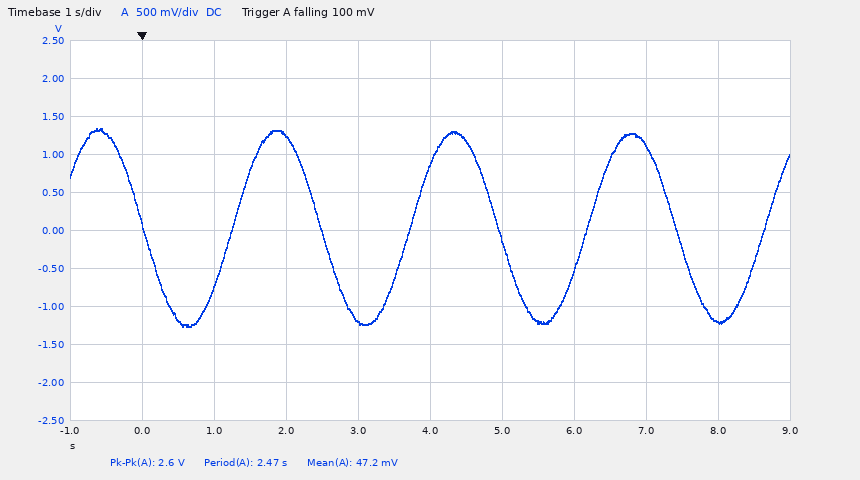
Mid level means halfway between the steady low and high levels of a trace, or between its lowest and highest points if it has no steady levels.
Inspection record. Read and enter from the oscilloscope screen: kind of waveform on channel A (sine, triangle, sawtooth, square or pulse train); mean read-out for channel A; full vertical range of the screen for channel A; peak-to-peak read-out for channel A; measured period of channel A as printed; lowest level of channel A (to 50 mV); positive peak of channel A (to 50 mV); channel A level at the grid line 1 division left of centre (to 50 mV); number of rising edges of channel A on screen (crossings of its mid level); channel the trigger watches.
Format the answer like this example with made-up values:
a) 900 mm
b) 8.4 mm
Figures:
a) sine
b) 47.2 mV
c) 5 V
d) 2.6 V
e) 2.47 s
f) -1.25 V
g) 1.35 V
h) -1.20 V
i) 4
j) channel A
